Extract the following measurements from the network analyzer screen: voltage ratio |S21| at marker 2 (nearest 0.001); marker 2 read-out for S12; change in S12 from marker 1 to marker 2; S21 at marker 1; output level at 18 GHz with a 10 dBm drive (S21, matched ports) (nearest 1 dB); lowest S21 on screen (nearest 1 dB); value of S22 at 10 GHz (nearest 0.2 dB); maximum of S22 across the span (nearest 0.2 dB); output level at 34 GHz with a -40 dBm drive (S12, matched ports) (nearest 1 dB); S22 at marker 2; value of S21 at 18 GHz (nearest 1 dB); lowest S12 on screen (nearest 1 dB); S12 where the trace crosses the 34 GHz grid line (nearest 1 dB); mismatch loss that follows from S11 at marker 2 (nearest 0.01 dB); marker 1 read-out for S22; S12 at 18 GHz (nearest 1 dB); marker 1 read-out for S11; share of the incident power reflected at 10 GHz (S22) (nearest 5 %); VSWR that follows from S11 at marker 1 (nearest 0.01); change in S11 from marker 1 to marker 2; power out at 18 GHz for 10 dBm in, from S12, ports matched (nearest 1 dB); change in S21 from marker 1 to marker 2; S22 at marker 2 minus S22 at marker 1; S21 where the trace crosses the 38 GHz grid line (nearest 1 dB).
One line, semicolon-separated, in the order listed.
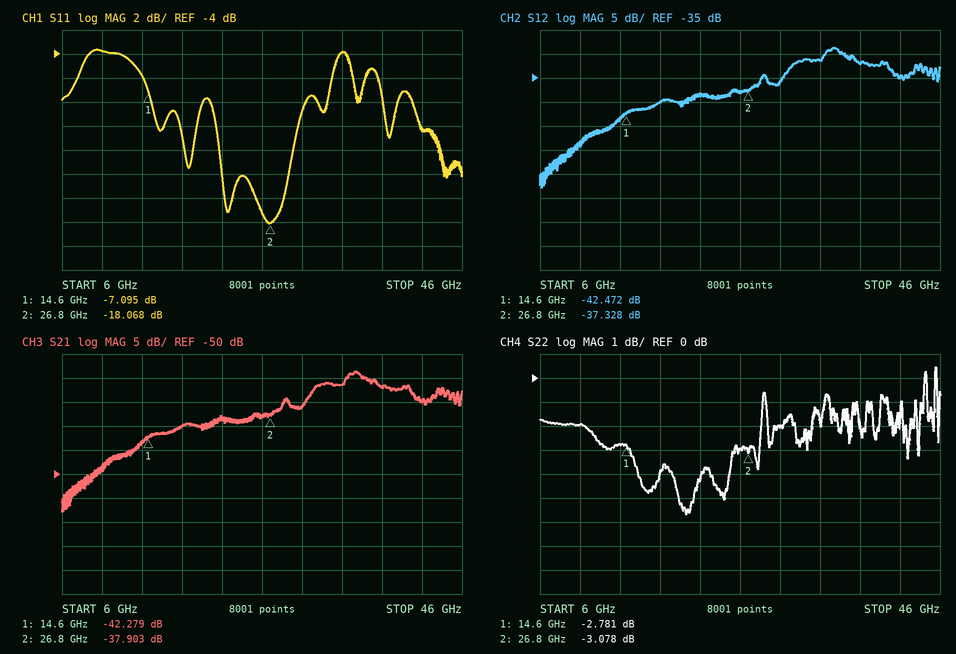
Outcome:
0.013; -37.328 dB; 5.144 dB; -42.279 dB; -30 dBm; -58 dB; -2.0 dB; 0.4 dB; -71 dBm; -3.078 dB; -40 dB; -58 dB; -31 dB; 0.07 dB; -2.781 dB; -40 dB; -7.095 dB; 65 %; 2.58; -10.973 dB; -30 dBm; 4.376 dB; -0.297 dB; -32 dB
